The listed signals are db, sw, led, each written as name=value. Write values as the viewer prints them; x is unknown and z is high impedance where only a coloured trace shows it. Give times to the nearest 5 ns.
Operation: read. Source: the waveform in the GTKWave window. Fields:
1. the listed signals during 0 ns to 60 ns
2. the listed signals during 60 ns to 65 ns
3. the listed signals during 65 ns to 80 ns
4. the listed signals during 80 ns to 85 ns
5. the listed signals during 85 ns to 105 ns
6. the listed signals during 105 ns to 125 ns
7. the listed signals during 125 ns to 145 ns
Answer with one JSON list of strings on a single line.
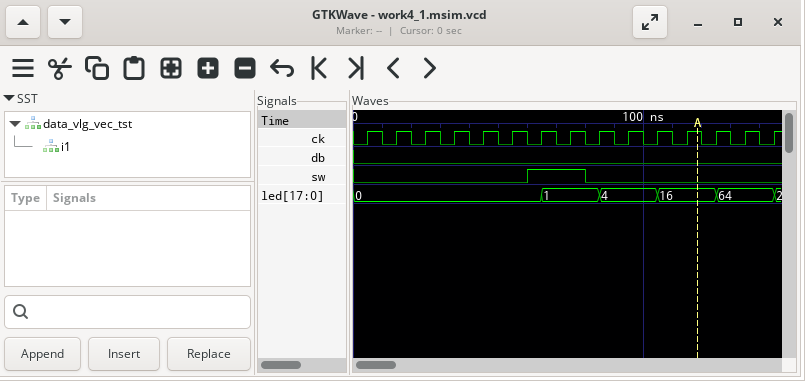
["db=0, sw=0, led=0", "db=0, sw=1, led=0", "db=0, sw=1, led=1", "db=0, sw=0, led=1", "db=0, sw=0, led=4", "db=0, sw=0, led=16", "db=0, sw=0, led=64"]
